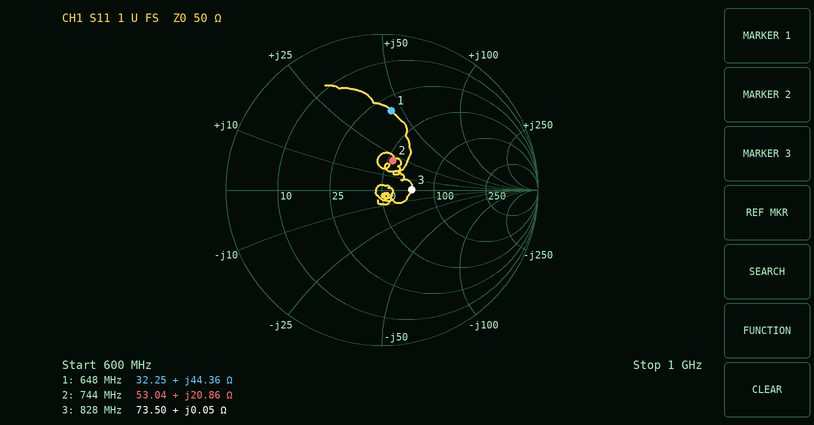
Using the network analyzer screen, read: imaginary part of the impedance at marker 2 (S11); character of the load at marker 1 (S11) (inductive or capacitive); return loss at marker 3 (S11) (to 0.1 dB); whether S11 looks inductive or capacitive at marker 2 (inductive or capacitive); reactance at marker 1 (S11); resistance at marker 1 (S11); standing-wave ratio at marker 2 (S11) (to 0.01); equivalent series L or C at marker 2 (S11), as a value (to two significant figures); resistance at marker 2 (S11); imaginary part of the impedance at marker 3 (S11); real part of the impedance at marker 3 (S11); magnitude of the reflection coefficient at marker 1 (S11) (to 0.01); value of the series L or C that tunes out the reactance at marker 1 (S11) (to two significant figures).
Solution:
+20.86 Ω
inductive
14.4 dB
inductive
+44.36 Ω
32.25 Ω
1.50
4.5 nH
53.04 Ω
+0.05 Ω
73.50 Ω
0.51
5.5 pF
